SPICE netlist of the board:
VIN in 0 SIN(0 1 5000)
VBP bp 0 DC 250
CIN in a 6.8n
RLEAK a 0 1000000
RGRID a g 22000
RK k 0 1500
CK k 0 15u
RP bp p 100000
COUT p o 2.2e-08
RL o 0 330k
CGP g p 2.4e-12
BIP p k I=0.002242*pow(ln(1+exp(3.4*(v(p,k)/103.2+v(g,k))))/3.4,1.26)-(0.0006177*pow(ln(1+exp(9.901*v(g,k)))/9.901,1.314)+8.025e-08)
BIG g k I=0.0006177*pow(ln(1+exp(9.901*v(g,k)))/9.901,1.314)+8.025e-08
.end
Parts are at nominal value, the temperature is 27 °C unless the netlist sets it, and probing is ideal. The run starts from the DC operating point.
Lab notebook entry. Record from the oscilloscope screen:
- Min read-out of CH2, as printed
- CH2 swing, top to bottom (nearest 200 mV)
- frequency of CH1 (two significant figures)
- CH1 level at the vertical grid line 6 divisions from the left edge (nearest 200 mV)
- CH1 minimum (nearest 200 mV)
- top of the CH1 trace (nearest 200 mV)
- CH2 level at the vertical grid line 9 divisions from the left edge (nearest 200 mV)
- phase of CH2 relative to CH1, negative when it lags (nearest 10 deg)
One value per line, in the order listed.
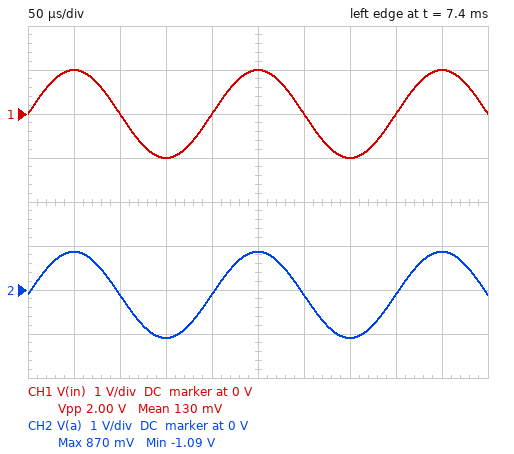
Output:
-1.09 V
2.0 V
5.0 kHz
0 V
-1.0 V
1.0 V
800 mV
0 deg
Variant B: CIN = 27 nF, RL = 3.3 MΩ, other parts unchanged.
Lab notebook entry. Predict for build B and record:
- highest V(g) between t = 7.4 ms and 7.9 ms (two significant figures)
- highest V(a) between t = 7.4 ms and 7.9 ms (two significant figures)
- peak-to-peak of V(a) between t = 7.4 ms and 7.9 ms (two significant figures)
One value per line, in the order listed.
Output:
880 mV
900 mV
2.0 V
